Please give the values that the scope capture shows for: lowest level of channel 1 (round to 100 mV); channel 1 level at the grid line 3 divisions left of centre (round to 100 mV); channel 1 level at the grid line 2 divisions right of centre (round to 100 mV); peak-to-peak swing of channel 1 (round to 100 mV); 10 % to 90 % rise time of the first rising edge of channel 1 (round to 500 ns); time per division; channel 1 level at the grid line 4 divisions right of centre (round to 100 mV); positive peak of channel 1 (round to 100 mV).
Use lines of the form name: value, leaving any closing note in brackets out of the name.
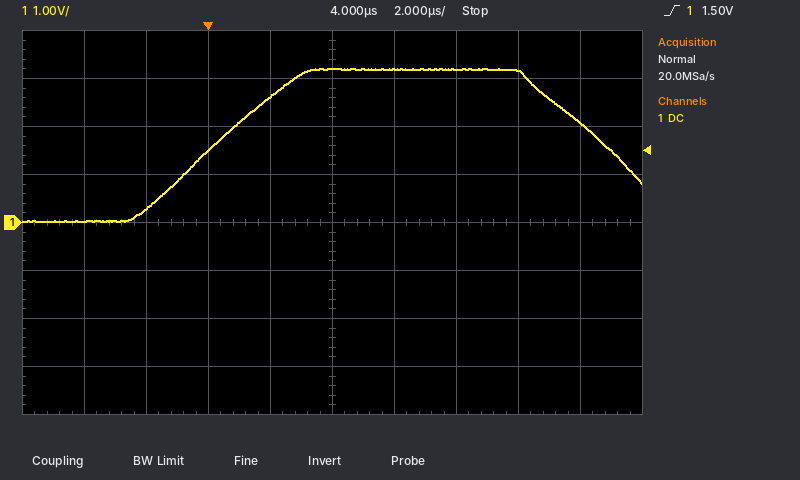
lowest level of channel 1: 0.0 V
channel 1 level at the grid line 3 divisions left of centre: 300 mV
channel 1 level at the grid line 2 divisions right of centre: 3.2 V
peak-to-peak swing of channel 1: 3.2 V
10 % to 90 % rise time of the first rising edge of channel 1: 4.5 µs
time per division: 2 µs
channel 1 level at the grid line 4 divisions right of centre: 2.1 V
positive peak of channel 1: 3.2 V
